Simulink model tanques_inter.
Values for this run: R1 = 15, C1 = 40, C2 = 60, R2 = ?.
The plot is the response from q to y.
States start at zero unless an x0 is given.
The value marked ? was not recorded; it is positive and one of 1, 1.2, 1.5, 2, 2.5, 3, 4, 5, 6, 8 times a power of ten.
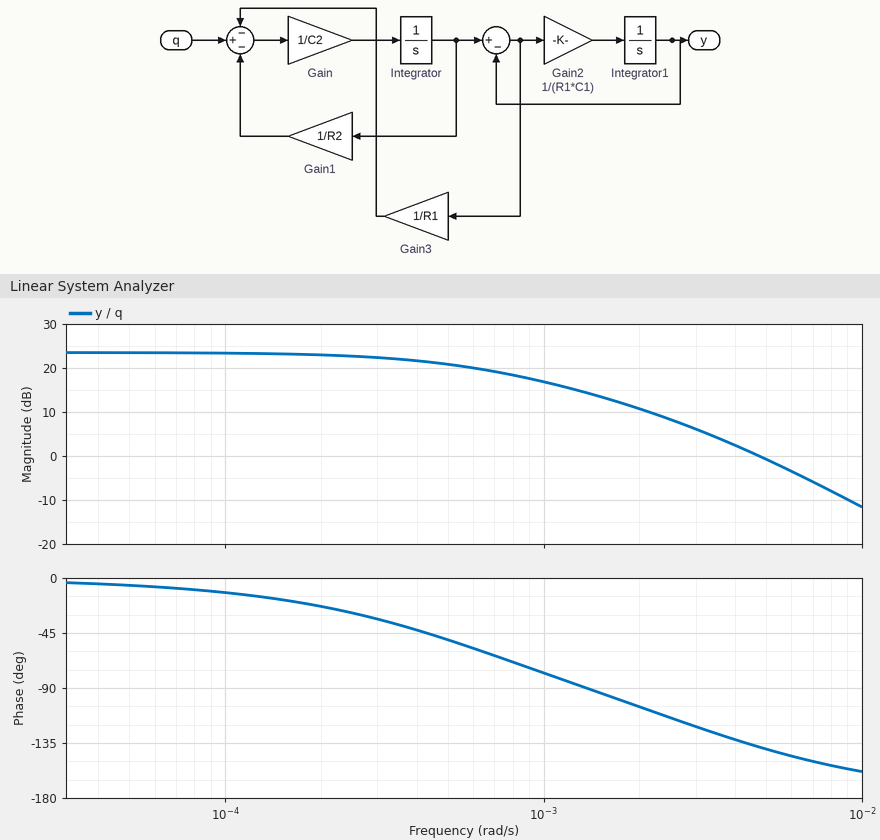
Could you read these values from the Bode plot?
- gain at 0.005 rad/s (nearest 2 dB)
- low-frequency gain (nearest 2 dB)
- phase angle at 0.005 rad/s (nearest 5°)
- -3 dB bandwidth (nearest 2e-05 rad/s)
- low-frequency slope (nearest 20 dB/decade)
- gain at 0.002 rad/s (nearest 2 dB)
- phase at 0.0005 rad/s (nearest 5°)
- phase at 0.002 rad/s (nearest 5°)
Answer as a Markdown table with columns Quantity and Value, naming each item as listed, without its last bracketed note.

| Quantity | Value |
|---|---|
| gain at 0.005 rad/s | 0 dB |
| low-frequency gain | 24 dB |
| phase angle at 0.005 rad/s | -140° |
| -3 dB bandwidth | 0.00054 rad/s |
| low-frequency slope | 0 dB/decade |
| gain at 0.002 rad/s | 10 dB |
| phase at 0.0005 rad/s | -50° |
| phase at 0.002 rad/s | -105° |
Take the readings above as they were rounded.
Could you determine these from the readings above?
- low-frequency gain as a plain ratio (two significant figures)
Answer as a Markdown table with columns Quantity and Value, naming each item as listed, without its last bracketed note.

| Quantity | Value |
|---|---|
| low-frequency gain as a plain ratio | 16 |
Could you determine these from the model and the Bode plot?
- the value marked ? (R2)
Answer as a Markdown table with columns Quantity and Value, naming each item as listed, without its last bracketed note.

| Quantity | Value |
|---|---|
| the value marked ? | 15 |
